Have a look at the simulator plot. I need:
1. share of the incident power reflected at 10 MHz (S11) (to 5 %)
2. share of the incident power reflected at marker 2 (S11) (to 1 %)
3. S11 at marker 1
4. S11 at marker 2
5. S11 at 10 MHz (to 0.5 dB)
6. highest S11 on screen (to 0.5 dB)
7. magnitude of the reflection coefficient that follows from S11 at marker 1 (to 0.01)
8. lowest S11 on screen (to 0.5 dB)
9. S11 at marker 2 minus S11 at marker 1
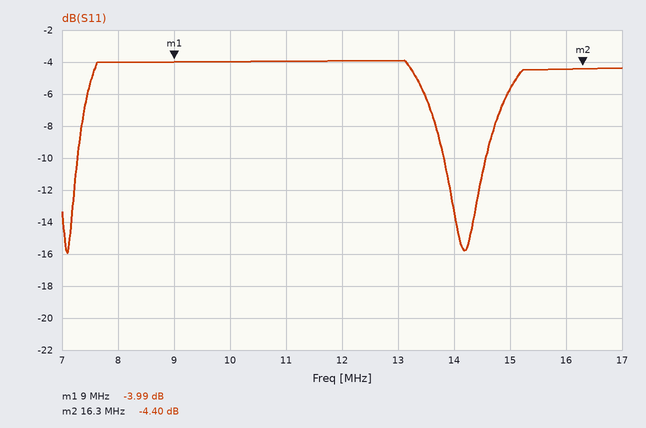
40 %
36 %
-3.99 dB
-4.40 dB
-4.0 dB
-4.0 dB
0.63
-16.0 dB
-0.41 dB
